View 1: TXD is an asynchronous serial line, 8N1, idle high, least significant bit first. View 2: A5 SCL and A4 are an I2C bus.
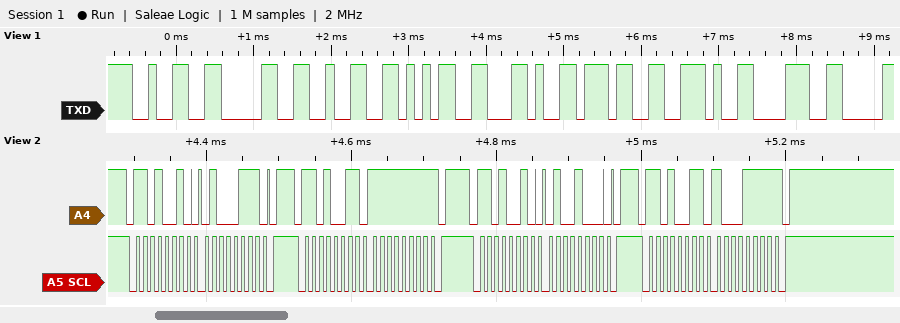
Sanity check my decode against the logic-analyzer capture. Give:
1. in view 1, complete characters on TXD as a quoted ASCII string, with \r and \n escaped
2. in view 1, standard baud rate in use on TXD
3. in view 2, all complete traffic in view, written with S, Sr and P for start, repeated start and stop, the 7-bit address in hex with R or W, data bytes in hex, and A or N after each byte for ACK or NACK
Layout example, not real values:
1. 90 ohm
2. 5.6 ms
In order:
1. "2025,7.8"
2. 9600 baud
3. S 69W A 47 A P S 69R A FF N P S 69W A 48 A P S 69R A 8F N P
